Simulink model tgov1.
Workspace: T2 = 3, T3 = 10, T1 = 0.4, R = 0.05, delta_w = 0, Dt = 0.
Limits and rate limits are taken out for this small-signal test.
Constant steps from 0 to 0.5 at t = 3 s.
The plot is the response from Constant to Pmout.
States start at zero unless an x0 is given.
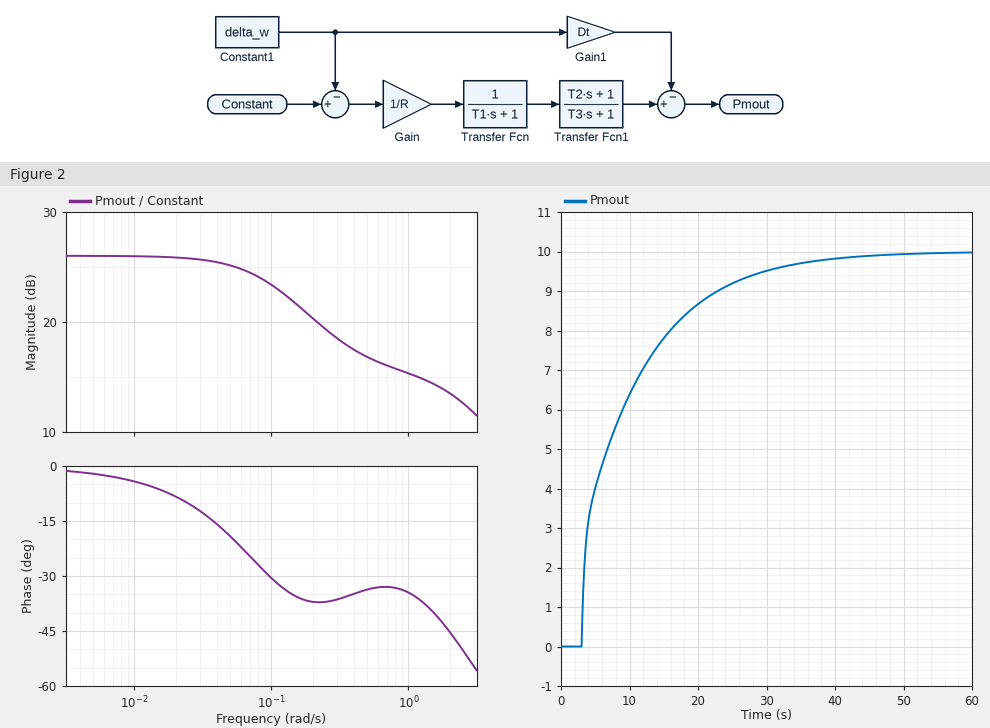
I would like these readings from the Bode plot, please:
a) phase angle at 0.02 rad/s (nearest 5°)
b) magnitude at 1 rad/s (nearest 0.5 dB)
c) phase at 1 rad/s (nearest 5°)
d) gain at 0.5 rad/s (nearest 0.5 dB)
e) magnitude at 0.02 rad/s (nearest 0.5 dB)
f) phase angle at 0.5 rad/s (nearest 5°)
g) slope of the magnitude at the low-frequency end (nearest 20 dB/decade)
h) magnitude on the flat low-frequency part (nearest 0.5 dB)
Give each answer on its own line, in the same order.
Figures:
-10°
15.5 dB
-35°
17.0 dB
26.0 dB
-35°
0 dB/decade
26.0 dB
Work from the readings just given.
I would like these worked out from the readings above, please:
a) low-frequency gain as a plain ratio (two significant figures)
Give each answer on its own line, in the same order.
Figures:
20
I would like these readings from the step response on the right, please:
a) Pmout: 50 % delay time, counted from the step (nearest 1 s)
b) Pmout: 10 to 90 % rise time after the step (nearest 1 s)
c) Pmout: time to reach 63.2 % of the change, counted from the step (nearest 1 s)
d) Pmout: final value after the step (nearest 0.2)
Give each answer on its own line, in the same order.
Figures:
4 s
20 s
7 s
10.0
